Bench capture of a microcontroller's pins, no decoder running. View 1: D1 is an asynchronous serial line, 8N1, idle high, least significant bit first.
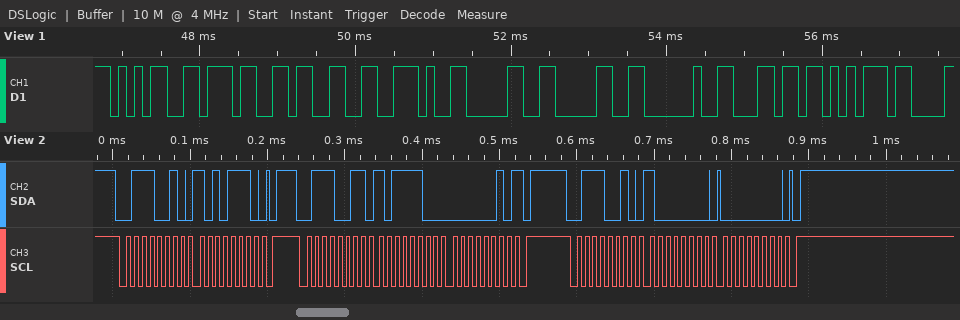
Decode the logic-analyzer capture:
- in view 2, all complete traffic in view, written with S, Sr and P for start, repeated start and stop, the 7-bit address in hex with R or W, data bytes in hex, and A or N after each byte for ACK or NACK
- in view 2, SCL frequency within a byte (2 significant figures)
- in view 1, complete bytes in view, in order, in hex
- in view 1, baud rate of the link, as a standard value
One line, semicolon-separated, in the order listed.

S 39W A AE A P S 39R A BC A 02 N P S 39W A 80 A 00 A P; 100 kHz; 0x35 0x37 0x33 0x2E 0x30 0x30 0x20 0x6C 0x75; 9600 baud
